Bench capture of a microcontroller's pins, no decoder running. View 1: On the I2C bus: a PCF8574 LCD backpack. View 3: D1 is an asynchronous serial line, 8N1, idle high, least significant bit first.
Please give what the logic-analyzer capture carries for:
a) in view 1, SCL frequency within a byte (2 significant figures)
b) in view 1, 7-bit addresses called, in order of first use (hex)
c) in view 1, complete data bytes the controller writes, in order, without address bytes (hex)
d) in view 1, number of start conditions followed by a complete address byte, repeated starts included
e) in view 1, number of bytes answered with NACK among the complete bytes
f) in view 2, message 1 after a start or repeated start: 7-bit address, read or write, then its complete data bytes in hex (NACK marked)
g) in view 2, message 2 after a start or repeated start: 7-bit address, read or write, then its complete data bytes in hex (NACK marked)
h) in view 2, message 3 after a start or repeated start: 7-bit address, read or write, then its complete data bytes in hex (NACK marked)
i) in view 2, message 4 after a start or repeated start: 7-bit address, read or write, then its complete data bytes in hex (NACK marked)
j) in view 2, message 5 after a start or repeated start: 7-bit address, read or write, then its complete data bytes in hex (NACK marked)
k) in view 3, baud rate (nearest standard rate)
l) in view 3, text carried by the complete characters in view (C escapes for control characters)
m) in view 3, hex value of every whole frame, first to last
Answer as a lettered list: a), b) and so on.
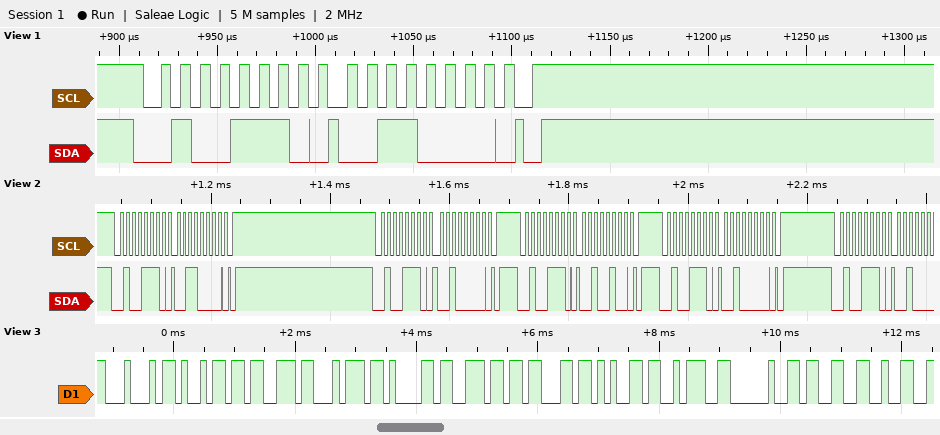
a) 100 kHz
b) 0x27
c) 30
d) 1
e) 0
f) 0x27 write: 30
g) 0x27 write: 20
h) 0x27 write: 24
i) 0x27 write: 20
j) 0x27 write
k) 9600 baud
l) "Distance: 32"
m) 44 69 73 74 61 6E 63 65 3A 20 33 32
